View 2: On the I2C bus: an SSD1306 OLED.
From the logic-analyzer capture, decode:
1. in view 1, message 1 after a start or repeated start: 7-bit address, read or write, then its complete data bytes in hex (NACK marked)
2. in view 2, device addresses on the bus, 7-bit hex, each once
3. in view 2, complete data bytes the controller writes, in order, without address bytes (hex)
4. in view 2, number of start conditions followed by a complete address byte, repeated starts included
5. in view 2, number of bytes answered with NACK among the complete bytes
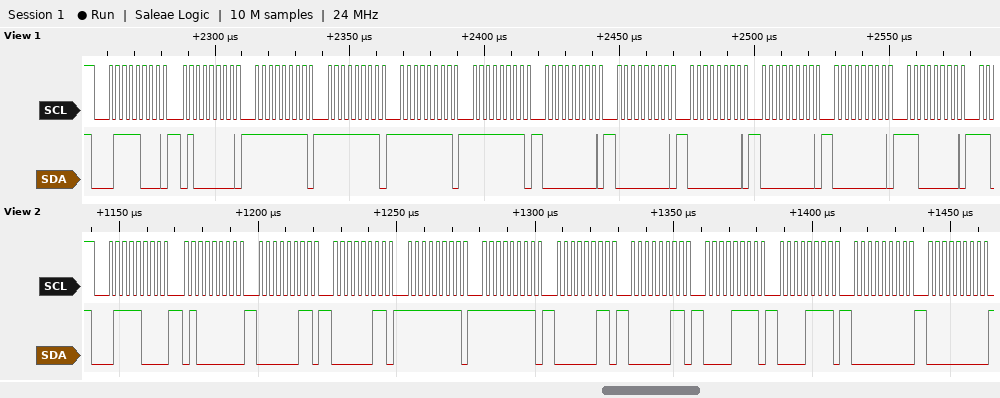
0x3C write: 40 FF FF FF FF 00 00 00 00 00 C0
0x3C
40 03 03 FF FF 03 03 0F 0F 00 00
1
0
